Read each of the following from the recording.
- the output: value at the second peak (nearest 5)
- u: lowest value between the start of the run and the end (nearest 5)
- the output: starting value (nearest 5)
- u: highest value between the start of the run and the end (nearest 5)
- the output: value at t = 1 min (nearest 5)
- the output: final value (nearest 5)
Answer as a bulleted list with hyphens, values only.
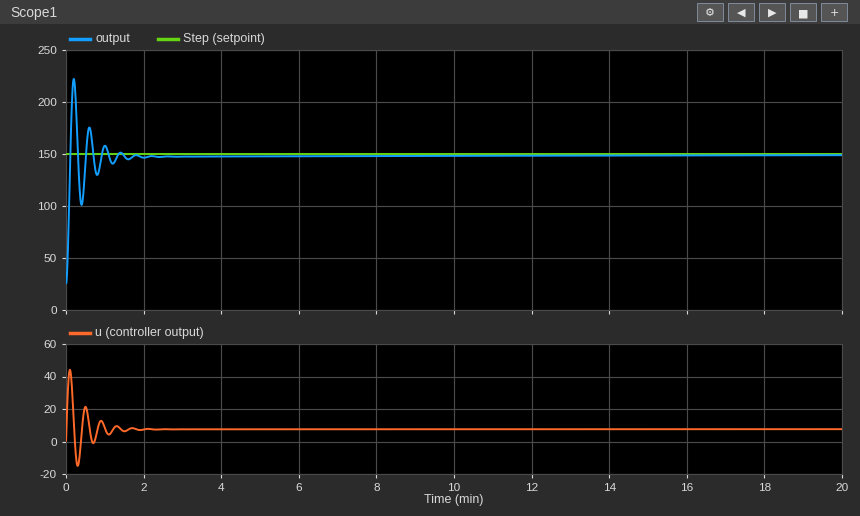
- 175
- -15
- 25
- 45
- 160
- 150
